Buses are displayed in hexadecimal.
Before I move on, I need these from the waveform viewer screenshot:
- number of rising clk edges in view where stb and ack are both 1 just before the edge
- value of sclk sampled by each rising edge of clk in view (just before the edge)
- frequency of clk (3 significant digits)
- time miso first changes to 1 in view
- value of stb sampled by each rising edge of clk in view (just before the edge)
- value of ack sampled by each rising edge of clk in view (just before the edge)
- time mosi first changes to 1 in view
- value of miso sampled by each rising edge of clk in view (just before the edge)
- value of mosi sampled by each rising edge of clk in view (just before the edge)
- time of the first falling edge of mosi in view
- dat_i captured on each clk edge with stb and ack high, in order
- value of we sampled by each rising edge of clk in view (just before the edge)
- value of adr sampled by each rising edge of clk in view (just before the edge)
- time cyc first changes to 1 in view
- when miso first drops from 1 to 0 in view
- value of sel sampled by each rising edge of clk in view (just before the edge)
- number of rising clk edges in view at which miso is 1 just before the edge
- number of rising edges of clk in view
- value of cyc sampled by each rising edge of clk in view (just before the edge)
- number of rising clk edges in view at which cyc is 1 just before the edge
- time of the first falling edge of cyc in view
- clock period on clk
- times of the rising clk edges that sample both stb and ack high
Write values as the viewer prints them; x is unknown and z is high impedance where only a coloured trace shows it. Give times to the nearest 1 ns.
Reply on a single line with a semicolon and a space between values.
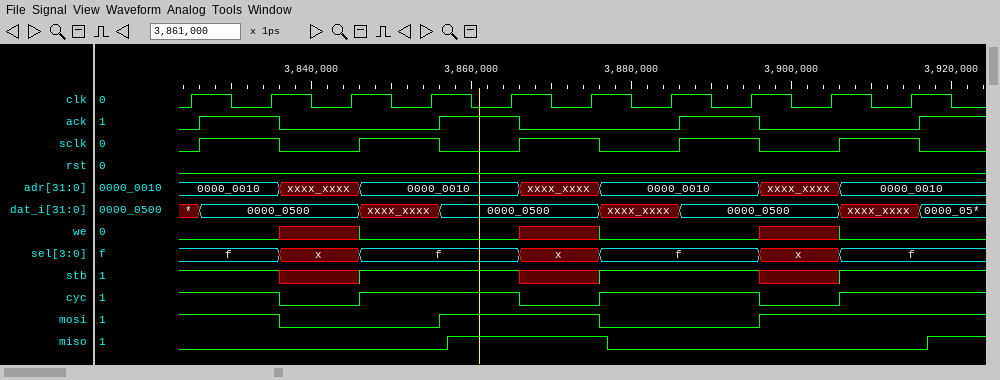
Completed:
3; 0 1 0 1 0 1 0 1 0 1; 100 MHz; 3857 ns; 1 1 x 1 1 x 1 1 x 1; 0 1 0 0 1 0 0 1 0 0; 3856 ns; 0 0 0 0 1 1 0 0 0 0; 1 1 0 0 1 1 0 0 1 1; 3836 ns; 0000_0500, 0000_0500, 0000_0500; 0 0 x 0 0 x 0 0 x 0; 0000_0010, 0000_0010, xxxx_xxxx, 0000_0010, 0000_0010, xxxx_xxxx, 0000_0010, 0000_0010, xxxx_xxxx, 0000_0010; 3846 ns; 3877 ns; f, f, x, f, f, x, f, f, x, f; 2; 10; 1 1 0 1 1 0 1 1 0 1; 7; 3836 ns; 10 ns; 3835 ns, 3865 ns, 3895 ns
